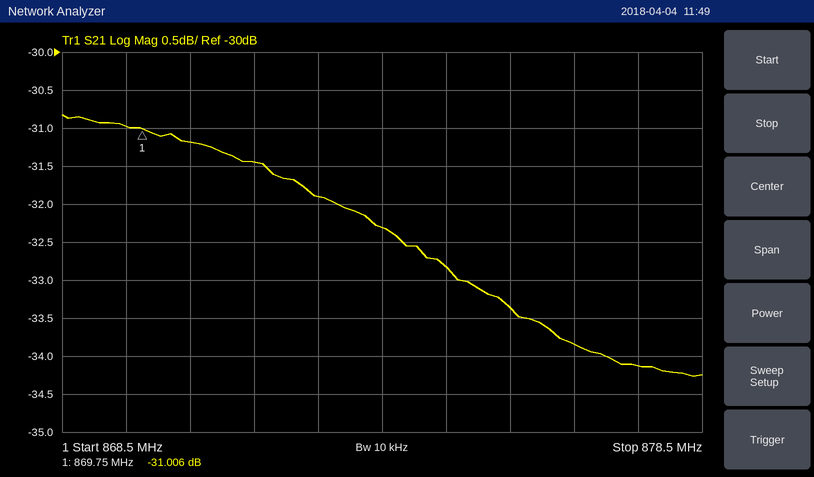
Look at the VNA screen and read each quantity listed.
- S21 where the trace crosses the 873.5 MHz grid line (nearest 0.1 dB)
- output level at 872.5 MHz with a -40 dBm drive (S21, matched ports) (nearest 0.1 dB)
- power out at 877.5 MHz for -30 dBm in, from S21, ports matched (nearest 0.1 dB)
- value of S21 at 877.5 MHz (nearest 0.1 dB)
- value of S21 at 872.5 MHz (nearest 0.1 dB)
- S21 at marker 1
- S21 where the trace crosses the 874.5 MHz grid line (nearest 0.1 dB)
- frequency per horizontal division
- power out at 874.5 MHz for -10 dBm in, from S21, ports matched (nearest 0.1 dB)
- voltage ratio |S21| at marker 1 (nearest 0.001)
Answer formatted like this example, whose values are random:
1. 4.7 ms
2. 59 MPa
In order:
1. -32.3 dB
2. -71.9 dBm
3. -64.1 dBm
4. -34.1 dB
5. -31.9 dB
6. -31.006 dB
7. -32.8 dB
8. 1 MHz
9. -42.8 dBm
10. 0.028
